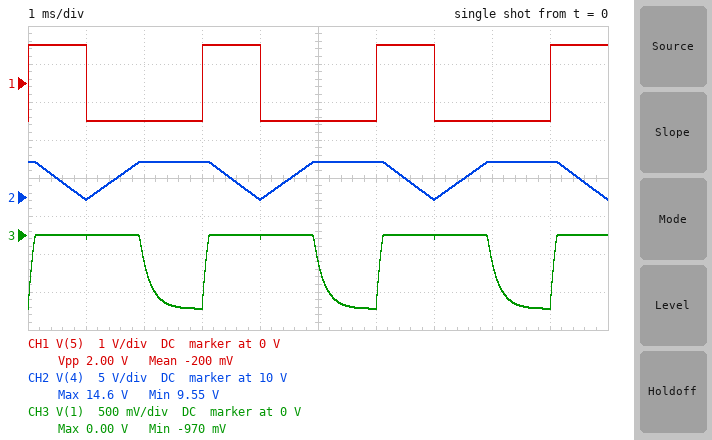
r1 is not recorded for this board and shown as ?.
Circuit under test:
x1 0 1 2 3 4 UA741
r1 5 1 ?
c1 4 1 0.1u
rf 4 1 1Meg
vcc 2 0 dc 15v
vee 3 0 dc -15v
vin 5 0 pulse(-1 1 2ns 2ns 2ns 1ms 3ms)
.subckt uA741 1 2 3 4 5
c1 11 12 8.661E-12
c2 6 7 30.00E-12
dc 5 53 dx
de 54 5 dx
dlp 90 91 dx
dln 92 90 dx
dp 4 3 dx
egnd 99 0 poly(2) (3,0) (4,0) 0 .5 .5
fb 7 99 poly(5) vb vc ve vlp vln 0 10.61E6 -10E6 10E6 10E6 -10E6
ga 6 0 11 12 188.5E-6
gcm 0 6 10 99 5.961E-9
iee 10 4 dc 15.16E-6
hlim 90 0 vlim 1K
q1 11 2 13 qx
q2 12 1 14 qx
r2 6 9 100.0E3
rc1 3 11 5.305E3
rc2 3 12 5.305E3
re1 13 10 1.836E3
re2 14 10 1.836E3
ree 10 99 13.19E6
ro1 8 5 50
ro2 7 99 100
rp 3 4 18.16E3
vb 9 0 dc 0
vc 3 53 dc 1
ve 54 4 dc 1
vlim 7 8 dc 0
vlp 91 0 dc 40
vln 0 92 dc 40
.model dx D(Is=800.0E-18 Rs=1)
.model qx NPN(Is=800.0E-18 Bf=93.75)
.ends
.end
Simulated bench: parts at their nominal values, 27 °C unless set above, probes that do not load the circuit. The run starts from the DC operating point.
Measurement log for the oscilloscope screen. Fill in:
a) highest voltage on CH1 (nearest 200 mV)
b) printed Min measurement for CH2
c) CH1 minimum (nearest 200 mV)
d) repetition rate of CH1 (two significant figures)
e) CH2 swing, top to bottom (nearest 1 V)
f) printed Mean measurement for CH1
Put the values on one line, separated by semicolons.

1.0 V; 9.55 V; -1.0 V; 330 Hz; 5 V; -200 mV
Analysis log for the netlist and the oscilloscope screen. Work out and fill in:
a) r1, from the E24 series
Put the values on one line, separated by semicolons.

1.8 kΩ
